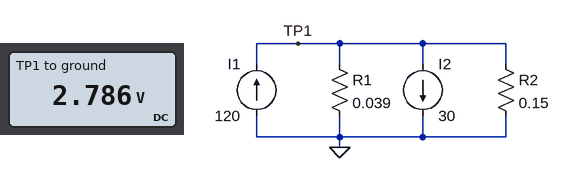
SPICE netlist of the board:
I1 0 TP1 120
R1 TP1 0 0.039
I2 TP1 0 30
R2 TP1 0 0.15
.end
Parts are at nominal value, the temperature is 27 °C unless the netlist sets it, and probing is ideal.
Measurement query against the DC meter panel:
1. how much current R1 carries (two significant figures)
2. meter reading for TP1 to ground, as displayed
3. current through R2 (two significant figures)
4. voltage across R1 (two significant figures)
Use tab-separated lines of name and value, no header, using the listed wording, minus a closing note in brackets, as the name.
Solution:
how much current R1 carries	71 A
meter reading for TP1 to ground, as displayed	2.786 V
current through R2	19 A
voltage across R1	2.8 V
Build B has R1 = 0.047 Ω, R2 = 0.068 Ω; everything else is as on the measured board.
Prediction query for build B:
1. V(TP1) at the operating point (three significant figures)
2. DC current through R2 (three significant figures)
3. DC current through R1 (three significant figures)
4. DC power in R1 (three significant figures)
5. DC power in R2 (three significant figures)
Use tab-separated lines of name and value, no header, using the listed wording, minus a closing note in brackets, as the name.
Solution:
V(TP1) at the operating point	2.50 V
DC current through R2	36.8 A
DC current through R1	53.2 A
DC power in R1	133 W
DC power in R2	92.0 W
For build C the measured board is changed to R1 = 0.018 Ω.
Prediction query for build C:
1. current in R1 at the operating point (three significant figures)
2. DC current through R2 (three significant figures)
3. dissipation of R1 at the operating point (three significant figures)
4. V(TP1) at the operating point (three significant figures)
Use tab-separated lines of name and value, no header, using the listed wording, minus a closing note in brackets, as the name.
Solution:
current in R1 at the operating point	80.4 A
DC current through R2	9.64 A
dissipation of R1 at the operating point	116 W
V(TP1) at the operating point	1.45 V
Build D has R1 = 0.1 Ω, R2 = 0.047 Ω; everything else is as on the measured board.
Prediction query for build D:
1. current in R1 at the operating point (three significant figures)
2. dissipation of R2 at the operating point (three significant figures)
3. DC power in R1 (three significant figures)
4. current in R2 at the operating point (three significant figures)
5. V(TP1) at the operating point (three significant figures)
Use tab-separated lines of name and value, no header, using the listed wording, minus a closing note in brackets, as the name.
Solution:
current in R1 at the operating point	28.8 A
dissipation of R2 at the operating point	176 W
DC power in R1	82.8 W
current in R2 at the operating point	61.2 A
V(TP1) at the operating point	2.88 V
